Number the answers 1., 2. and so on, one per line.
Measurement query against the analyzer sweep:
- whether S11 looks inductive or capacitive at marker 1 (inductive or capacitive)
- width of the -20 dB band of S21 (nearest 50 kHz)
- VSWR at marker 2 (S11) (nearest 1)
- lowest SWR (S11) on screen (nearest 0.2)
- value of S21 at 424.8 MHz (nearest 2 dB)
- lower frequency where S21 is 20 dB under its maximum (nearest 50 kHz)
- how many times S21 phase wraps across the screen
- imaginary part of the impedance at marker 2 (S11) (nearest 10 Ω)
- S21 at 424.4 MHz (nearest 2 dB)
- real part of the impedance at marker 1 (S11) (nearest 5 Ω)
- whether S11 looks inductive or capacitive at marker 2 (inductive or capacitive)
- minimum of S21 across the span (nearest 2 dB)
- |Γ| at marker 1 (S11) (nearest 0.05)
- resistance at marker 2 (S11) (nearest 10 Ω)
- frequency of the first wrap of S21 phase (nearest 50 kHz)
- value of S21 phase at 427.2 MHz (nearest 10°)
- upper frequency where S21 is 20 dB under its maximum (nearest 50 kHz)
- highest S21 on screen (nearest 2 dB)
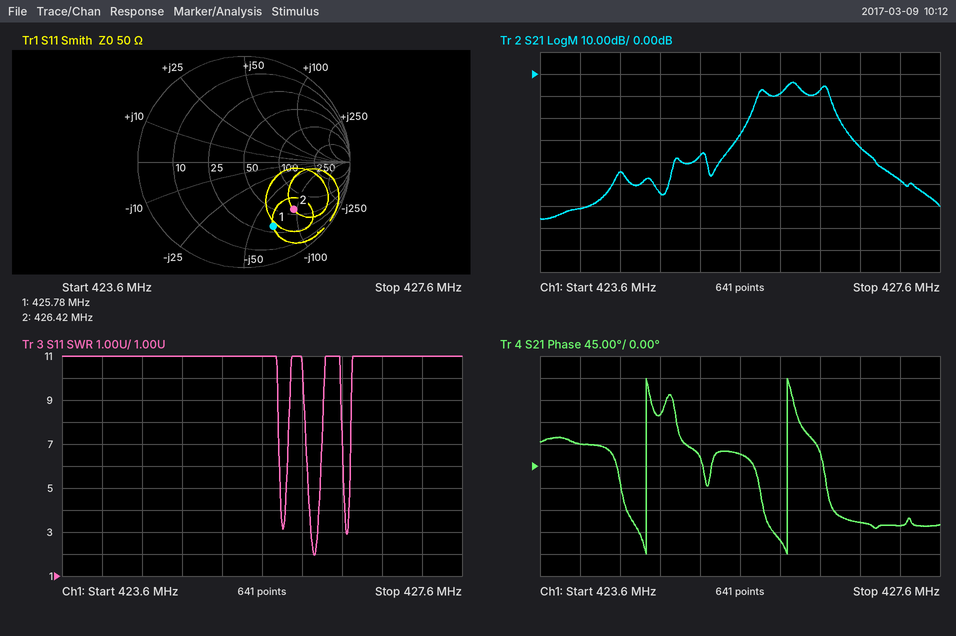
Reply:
1. capacitive
2. 1.00 MHz
3. 5
4. 2.0
5. -54 dB
6. 425.65 MHz
7. 2
8. -90 Ω
9. -44 dB
10. 30 Ω
11. capacitive
12. -66 dB
13. 0.65
14. 60 Ω
15. 424.65 MHz
16. -120°
17. 426.65 MHz
18. -4 dB
